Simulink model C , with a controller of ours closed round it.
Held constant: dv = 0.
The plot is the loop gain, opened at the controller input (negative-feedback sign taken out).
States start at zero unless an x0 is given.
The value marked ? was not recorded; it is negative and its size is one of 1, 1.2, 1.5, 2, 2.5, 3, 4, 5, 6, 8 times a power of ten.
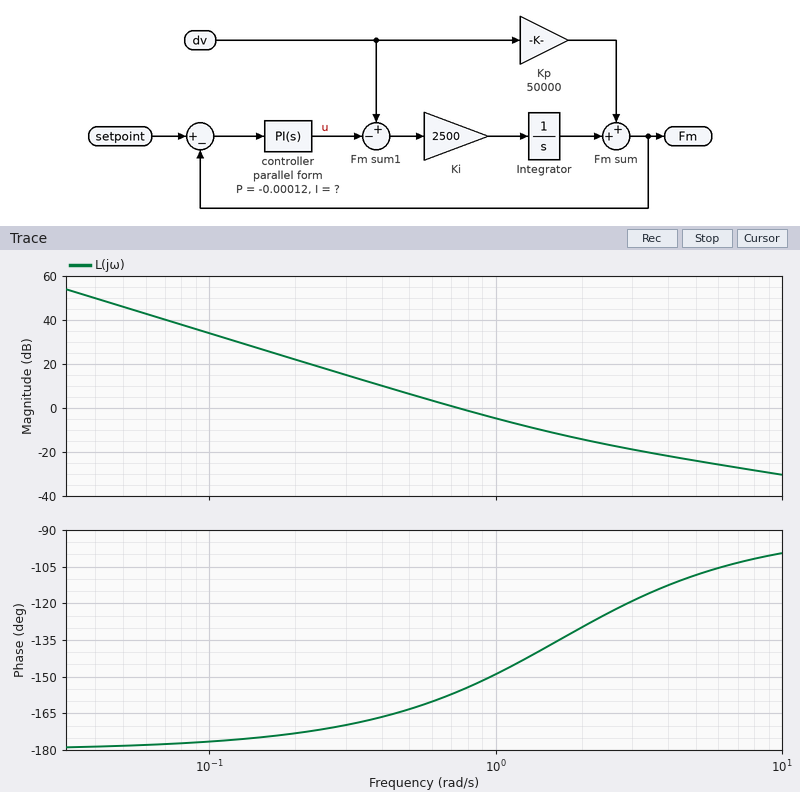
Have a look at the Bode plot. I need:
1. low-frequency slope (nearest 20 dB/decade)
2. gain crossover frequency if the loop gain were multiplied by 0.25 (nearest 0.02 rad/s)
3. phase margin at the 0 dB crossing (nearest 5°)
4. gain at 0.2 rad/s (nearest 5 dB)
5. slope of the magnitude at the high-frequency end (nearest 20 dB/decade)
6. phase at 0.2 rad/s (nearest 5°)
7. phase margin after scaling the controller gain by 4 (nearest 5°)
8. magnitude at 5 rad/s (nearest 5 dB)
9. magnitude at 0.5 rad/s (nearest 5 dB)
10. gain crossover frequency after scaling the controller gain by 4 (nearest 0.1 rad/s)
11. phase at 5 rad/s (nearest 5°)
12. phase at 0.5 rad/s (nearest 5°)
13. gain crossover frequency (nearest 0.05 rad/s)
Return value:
-40 dB/decade
0.36 rad/s
25°
20 dB
-20 dB/decade
-175°
45°
-25 dB
5 dB
1.7 rad/s
-110°
-165°
0.75 rad/s
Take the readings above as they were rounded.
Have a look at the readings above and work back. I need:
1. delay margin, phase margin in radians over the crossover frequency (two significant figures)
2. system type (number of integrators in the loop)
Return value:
0.58 s
2
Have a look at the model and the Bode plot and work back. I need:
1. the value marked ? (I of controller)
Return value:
-0.0002
